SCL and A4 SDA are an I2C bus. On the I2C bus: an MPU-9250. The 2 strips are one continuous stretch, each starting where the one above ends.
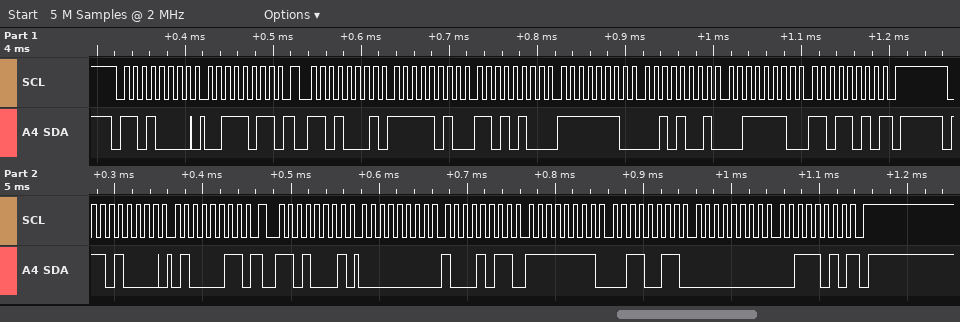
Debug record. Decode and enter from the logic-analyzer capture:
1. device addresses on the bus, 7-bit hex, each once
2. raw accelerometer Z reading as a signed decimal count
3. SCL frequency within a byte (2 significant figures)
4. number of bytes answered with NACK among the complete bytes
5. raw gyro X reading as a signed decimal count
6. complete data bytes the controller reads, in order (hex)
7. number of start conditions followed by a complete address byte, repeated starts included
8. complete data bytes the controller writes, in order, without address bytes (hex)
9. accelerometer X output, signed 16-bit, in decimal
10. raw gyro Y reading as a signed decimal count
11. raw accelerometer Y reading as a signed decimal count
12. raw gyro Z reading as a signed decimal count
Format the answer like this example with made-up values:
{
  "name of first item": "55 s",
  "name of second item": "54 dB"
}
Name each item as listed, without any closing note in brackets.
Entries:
{
  "device addresses on the bus, 7-bit hex, each once": "0x68",
  "raw accelerometer Z reading as a signed decimal count": "16090",
  "SCL frequency within a byte": "100 kHz",
  "number of bytes answered with NACK among the complete bytes": "2",
  "raw gyro X reading as a signed decimal count": "139",
  "complete data bytes the controller reads, in order": "FA D4 FE 29 3E DA 00 8B FF 33 00 3A",
  "number of start conditions followed by a complete address byte, repeated starts included": "4",
  "complete data bytes the controller writes, in order, without address bytes": "3B 43",
  "accelerometer X output, signed 16-bit, in decimal": "-1324",
  "raw gyro Y reading as a signed decimal count": "-205",
  "raw accelerometer Y reading as a signed decimal count": "-471",
  "raw gyro Z reading as a signed decimal count": "58"
}
